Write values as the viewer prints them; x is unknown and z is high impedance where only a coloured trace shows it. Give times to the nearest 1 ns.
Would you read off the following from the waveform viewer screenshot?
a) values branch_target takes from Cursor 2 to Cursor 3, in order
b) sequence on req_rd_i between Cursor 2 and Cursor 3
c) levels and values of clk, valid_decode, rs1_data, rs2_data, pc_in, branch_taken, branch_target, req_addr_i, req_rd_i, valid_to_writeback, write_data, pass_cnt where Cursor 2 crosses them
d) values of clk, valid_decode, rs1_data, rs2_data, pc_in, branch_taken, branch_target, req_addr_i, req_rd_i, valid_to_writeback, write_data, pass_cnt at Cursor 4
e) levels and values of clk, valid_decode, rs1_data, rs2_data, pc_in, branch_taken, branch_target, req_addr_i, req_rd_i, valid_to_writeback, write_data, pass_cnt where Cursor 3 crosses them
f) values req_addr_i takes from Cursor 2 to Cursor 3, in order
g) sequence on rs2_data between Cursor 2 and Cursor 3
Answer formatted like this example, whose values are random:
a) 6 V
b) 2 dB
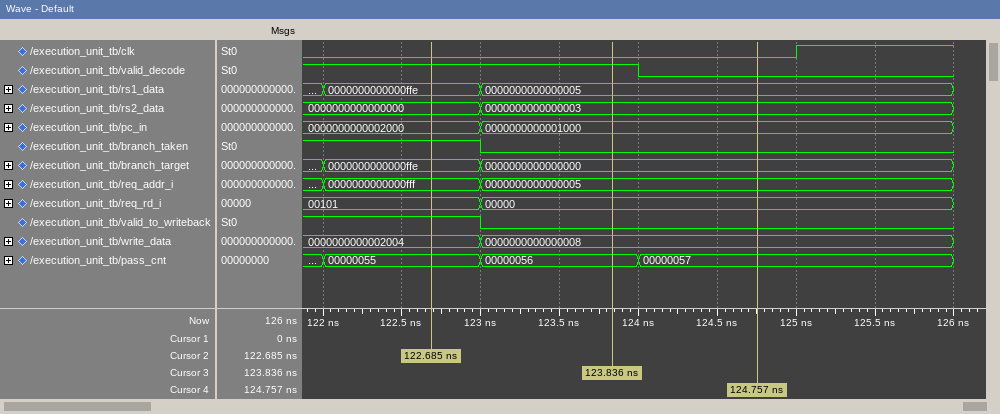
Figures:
a) 0000000000000ffe, 0000000000000000
b) 00101, 00000
c) clk=0, valid_decode=1, rs1_data=0000000000000ffe, rs2_data=0000000000000000, pc_in=0000000000002000, branch_taken=1, branch_target=0000000000000ffe, req_addr_i=0000000000000fff, req_rd_i=00101, valid_to_writeback=1, write_data=0000000000002004, pass_cnt=00000055
d) clk=0, valid_decode=0, rs1_data=0000000000000005, rs2_data=0000000000000003, pc_in=0000000000001000, branch_taken=0, branch_target=0000000000000000, req_addr_i=0000000000000005, req_rd_i=00000, valid_to_writeback=0, write_data=0000000000000008, pass_cnt=00000057
e) clk=0, valid_decode=1, rs1_data=0000000000000005, rs2_data=0000000000000003, pc_in=0000000000001000, branch_taken=0, branch_target=0000000000000000, req_addr_i=0000000000000005, req_rd_i=00000, valid_to_writeback=0, write_data=0000000000000008, pass_cnt=00000056
f) 0000000000000fff, 0000000000000005
g) 0000000000000000, 0000000000000003
